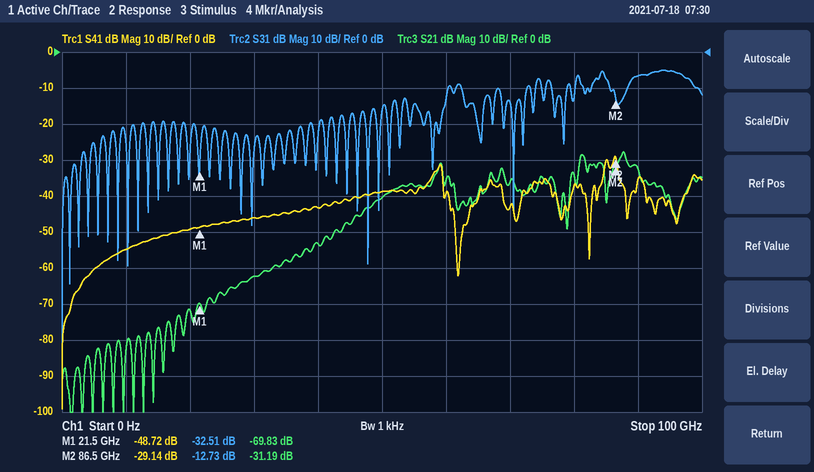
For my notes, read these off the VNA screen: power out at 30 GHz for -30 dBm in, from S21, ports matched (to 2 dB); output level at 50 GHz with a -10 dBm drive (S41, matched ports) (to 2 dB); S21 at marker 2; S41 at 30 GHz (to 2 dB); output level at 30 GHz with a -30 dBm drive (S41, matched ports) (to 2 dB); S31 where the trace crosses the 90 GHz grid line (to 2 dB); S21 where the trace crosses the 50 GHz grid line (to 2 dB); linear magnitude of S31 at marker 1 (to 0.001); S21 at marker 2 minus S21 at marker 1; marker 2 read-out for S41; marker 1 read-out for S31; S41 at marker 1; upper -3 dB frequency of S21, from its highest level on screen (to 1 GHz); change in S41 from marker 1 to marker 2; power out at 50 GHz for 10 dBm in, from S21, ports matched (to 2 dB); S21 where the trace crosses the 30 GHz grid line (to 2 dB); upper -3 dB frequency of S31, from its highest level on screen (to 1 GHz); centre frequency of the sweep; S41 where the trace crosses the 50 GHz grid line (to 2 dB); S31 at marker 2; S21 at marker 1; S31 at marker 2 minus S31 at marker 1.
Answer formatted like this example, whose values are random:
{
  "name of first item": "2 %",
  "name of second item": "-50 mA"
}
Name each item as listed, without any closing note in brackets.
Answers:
{
  "power out at 30 GHz for -30 dBm in, from S21, ports matched": "-92 dBm",
  "output level at 50 GHz with a -10 dBm drive (S41, matched ports)": "-48 dBm",
  "S21 at marker 2": "-31.19 dB",
  "S41 at 30 GHz": "-46 dB",
  "output level at 30 GHz with a -30 dBm drive (S41, matched ports)": "-76 dBm",
  "S31 where the trace crosses the 90 GHz grid line": "-6 dB",
  "S21 where the trace crosses the 50 GHz grid line": "-40 dB",
  "linear magnitude of S31 at marker 1": "0.024",
  "S21 at marker 2 minus S21 at marker 1": "38.64 dB",
  "marker 2 read-out for S41": "-29.14 dB",
  "marker 1 read-out for S31": "-32.51 dB",
  "S41 at marker 1": "-48.72 dB",
  "upper -3 dB frequency of S21, from its highest level on screen": "88 GHz",
  "change in S41 from marker 1 to marker 2": "19.58 dB",
  "power out at 50 GHz for 10 dBm in, from S21, ports matched": "-30 dBm",
  "S21 where the trace crosses the 30 GHz grid line": "-62 dB",
  "upper -3 dB frequency of S31, from its highest level on screen": "98 GHz",
  "centre frequency of the sweep": "50 GHz",
  "S41 where the trace crosses the 50 GHz grid line": "-38 dB",
  "S31 at marker 2": "-12.73 dB",
  "S21 at marker 1": "-69.83 dB",
  "S31 at marker 2 minus S31 at marker 1": "19.78 dB"
}
